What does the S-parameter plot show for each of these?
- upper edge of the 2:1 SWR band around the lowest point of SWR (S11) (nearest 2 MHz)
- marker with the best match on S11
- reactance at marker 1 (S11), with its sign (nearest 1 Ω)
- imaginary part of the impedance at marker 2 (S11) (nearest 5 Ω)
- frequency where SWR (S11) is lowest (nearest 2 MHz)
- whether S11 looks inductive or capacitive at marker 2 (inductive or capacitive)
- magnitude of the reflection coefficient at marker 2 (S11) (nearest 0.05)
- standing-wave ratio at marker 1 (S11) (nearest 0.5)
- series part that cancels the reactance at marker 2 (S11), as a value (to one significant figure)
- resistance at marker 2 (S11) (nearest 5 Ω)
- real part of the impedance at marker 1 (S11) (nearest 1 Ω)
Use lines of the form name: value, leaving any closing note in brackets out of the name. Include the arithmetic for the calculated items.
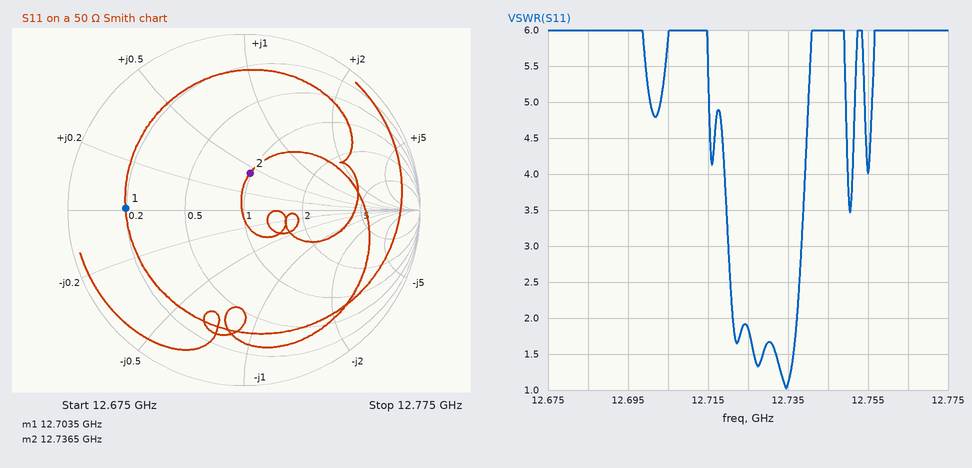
upper edge of the 2:1 SWR band around the lowest point of SWR (S11): 12.738 GHz
marker with the best match on S11: marker 2
reactance at marker 1 (S11), with its sign: 0 Ω
imaginary part of the impedance at marker 2 (S11): +20 Ω
frequency where SWR (S11) is lowest: 12.734 GHz
whether S11 looks inductive or capacitive at marker 2: inductive
magnitude of the reflection coefficient at marker 2 (S11): 0.20
standing-wave ratio at marker 1 (S11): 5.0
series part that cancels the reactance at marker 2 (S11), as a value: C = 1/(2π × 12.7365 GHz × 20 Ω) ≈ 625 fF, so 600 fF to one significant figure
resistance at marker 2 (S11): 50 Ω
real part of the impedance at marker 1 (S11): 10 Ω
